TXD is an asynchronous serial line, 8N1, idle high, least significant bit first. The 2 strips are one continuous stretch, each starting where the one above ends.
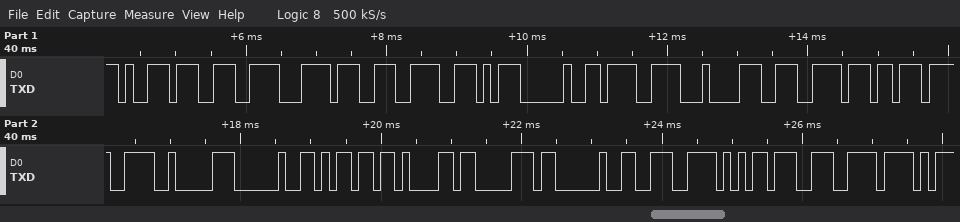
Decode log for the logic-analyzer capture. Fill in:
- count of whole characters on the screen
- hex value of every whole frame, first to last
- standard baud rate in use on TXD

21
0xB9 0xCE 0xBC 0xCE 0xAE 0x20 0xCF 0x84 0xCE 0xB7 0xCF 0x82 0x20 0x6D 0x61 0x70 0x20 0xCE 0xB5 0xCE 0xAF
9600 baud
